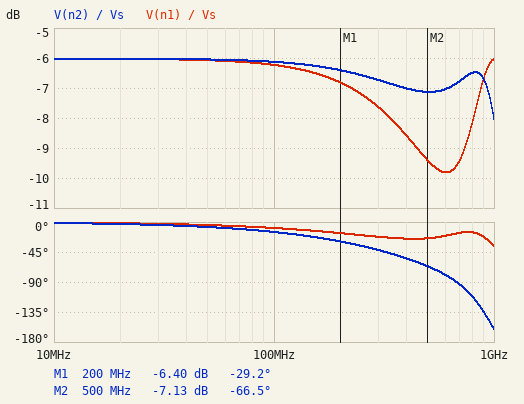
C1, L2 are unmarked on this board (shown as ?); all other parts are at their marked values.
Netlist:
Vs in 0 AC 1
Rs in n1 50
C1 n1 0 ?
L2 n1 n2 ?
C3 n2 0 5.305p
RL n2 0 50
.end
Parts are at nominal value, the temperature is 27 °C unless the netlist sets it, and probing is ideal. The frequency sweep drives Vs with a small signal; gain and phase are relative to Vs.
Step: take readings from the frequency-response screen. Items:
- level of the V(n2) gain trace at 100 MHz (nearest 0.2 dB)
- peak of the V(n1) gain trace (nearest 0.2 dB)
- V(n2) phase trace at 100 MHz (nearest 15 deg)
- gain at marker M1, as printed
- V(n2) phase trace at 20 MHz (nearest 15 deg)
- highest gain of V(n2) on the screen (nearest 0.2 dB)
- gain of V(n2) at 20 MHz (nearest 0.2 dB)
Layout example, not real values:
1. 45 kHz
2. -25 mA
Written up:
1. -6.2 dB
2. -6.0 dB
3. -15 deg
4. -6.40 dB
5. 0 deg
6. -6.0 dB
7. -6.0 dB
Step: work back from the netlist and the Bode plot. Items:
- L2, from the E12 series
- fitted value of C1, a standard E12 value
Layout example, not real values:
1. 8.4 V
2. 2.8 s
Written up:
1. 8.2 nH
2. 8.2 pF
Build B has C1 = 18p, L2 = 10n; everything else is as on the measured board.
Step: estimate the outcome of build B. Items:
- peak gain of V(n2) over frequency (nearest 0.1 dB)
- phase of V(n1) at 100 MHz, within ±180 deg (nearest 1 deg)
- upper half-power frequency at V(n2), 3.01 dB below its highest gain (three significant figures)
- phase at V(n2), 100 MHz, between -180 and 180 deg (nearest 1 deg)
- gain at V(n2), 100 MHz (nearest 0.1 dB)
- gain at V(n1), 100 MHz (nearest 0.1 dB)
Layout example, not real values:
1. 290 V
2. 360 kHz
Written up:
1. -6.0 dB
2. -17 deg
3. 506 MHz
4. -24 deg
5. -6.4 dB
6. -6.5 dB
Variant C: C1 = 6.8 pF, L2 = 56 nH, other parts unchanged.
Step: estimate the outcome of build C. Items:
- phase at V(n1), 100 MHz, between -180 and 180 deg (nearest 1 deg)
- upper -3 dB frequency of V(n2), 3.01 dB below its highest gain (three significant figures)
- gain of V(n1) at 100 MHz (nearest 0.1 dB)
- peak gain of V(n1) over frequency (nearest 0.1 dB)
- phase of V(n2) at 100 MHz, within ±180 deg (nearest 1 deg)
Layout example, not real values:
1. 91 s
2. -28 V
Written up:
1. 7 deg
2. 330 MHz
3. -5.1 dB
4. -1.6 dB
5. -31 deg
